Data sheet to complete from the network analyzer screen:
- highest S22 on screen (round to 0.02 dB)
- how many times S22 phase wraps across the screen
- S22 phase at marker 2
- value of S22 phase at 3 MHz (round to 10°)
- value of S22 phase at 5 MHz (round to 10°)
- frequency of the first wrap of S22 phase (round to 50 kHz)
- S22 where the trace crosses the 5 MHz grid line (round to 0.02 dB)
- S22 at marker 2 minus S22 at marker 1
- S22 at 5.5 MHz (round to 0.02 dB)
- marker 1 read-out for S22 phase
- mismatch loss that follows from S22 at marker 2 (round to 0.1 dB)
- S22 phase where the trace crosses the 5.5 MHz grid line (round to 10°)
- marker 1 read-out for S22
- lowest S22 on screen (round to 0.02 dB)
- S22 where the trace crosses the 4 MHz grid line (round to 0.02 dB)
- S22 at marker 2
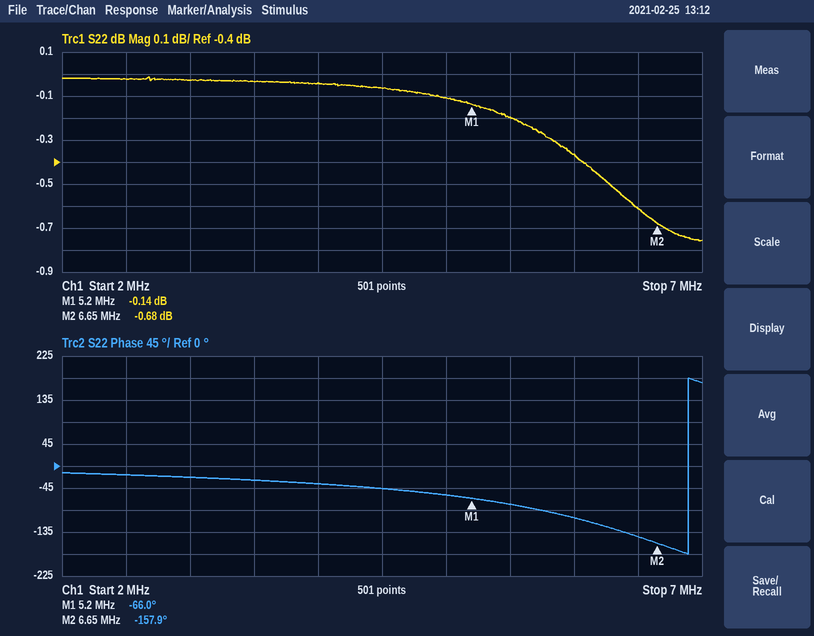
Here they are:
-0.02 dB
1
-157.9°
-20°
-60°
6.90 MHz
-0.10 dB
-0.54 dB
-0.20 dB
-66.0°
8.4 dB
-80°
-0.14 dB
-0.76 dB
-0.04 dB
-0.68 dB
